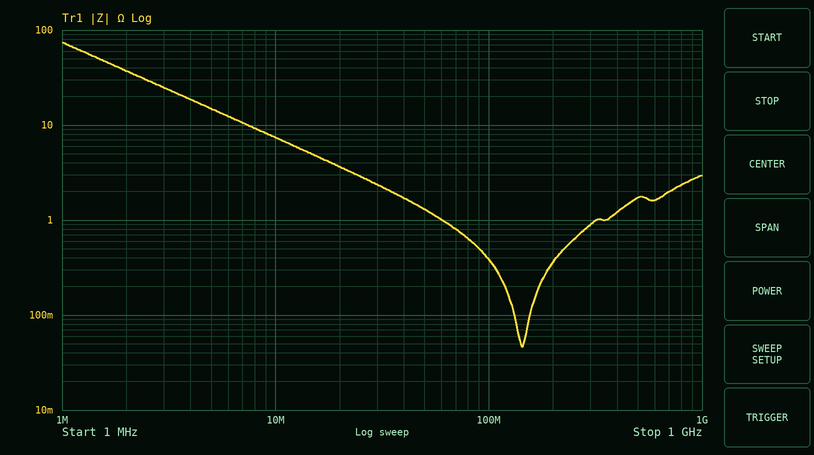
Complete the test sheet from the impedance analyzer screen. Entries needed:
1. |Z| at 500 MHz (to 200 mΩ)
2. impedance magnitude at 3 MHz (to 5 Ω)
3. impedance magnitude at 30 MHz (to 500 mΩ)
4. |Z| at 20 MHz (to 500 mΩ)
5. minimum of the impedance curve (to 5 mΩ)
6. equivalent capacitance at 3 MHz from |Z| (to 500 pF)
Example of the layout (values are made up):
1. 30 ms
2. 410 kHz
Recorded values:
1. 1.8 Ω
2. 25 Ω
3. 2.5 Ω
4. 3.5 Ω
5. 45 mΩ
6. 2.0 nF
